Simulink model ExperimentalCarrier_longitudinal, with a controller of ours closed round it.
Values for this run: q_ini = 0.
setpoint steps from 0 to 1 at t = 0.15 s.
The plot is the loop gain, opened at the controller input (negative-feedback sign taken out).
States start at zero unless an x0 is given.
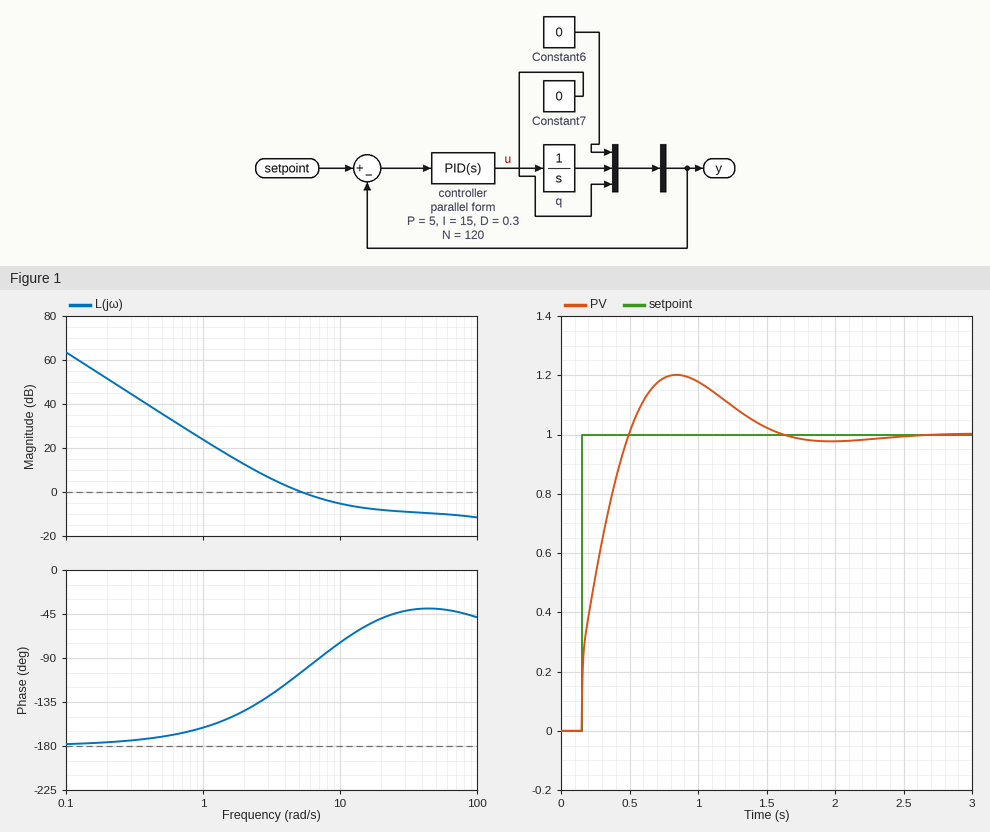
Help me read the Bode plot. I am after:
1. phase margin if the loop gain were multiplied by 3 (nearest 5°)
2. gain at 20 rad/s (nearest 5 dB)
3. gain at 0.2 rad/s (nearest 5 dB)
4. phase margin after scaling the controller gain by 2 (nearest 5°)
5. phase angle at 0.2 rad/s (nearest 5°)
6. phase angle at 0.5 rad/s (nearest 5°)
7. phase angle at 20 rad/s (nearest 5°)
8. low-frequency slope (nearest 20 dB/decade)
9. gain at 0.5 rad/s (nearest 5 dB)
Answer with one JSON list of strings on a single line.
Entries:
["140°", "-10 dB", "50 dB", "110°", "-175°", "-170°", "-50°", "-40 dB/decade", "35 dB"]
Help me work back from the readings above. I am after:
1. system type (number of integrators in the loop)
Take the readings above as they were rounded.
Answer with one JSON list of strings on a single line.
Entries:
["2"]
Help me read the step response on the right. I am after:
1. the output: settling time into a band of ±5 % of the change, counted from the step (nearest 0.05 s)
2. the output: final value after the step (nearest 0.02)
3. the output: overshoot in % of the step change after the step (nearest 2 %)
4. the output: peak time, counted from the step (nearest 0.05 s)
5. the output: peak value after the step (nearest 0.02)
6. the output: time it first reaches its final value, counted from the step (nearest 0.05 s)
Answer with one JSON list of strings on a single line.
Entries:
["1.25 s", "1.00", "20 %", "0.70 s", "1.20", "0.35 s"]
